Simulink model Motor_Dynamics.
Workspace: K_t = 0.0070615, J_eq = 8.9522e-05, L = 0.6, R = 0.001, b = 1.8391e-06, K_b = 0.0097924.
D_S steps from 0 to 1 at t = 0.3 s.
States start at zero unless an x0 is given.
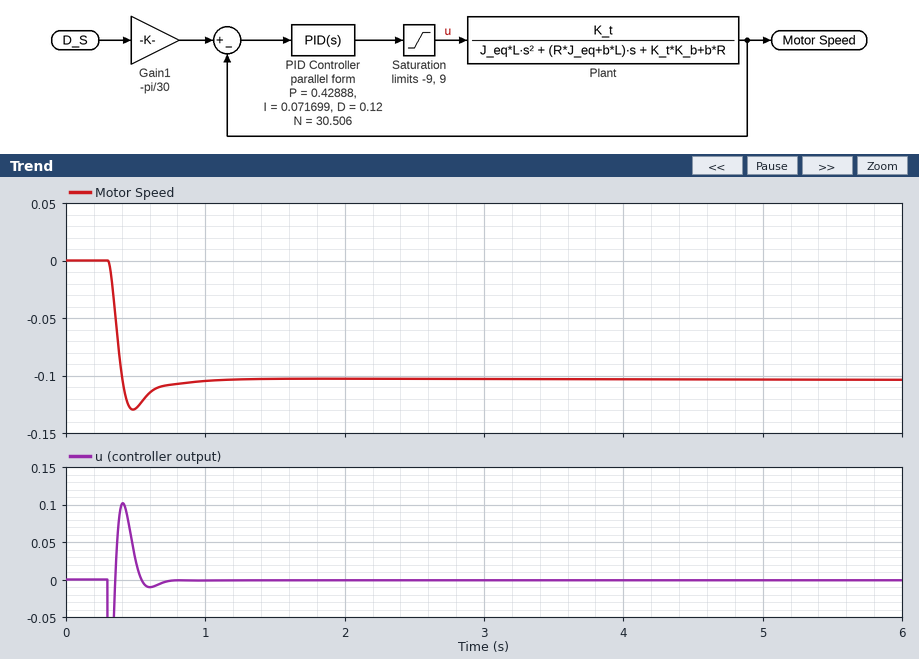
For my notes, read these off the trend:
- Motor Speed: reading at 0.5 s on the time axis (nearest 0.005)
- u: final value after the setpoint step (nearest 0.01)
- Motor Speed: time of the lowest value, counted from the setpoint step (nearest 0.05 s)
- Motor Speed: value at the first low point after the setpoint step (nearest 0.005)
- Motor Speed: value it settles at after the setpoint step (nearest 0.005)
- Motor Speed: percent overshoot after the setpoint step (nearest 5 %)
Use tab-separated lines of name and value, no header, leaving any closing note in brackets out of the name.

Motor Speed: reading at 0.5 s on the time axis	-0.130
u: final value after the setpoint step	0.00
Motor Speed: time of the lowest value, counted from the setpoint step	0.20 s
Motor Speed: value at the first low point after the setpoint step	-0.130
Motor Speed: value it settles at after the setpoint step	-0.105
Motor Speed: percent overshoot after the setpoint step	25 %
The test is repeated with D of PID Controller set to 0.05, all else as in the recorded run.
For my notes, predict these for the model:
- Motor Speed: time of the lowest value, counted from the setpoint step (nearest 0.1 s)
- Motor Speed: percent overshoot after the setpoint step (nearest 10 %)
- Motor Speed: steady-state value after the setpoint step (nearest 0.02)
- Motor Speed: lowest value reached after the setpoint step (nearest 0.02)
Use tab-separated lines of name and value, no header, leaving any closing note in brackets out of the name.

Motor Speed: time of the lowest value, counted from the setpoint step	0.3 s
Motor Speed: percent overshoot after the setpoint step	40 %
Motor Speed: steady-state value after the setpoint step	-0.10
Motor Speed: lowest value reached after the setpoint step	-0.14
